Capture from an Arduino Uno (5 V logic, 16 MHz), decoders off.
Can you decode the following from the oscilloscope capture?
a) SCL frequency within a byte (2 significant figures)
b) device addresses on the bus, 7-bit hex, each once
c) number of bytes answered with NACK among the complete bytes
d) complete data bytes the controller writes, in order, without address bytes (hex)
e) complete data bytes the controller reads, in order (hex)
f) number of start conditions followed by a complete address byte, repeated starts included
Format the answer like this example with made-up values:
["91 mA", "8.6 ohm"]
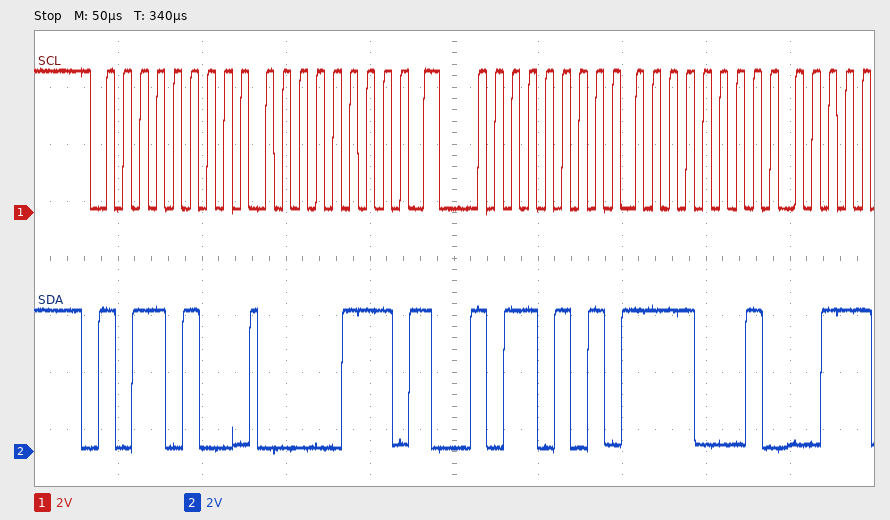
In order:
["100 kHz", "0x5A", "0", "07", "F1", "2"]
